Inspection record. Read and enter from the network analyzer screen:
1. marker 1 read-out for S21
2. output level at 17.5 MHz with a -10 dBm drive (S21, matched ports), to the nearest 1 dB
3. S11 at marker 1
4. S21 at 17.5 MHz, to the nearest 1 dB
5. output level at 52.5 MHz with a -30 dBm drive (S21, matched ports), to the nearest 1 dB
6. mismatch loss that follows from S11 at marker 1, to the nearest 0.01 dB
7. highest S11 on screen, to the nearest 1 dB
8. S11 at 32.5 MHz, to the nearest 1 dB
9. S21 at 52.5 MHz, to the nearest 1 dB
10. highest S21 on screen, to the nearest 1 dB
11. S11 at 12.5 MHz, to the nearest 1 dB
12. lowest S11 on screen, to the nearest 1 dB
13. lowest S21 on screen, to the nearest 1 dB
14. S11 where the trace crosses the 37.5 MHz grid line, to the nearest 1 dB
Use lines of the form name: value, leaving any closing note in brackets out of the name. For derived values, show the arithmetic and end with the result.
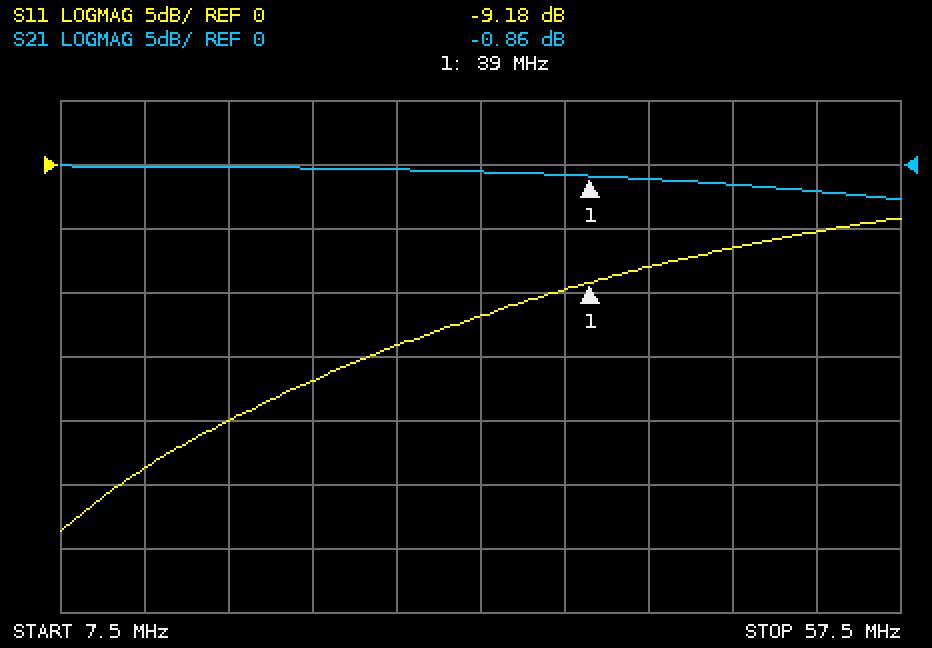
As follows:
marker 1 read-out for S21: -0.86 dB
output level at 17.5 MHz with a -10 dBm drive (S21, matched ports), to the nearest 1 dB: -10 dBm + (0 dB) = -10 dBm
S11 at marker 1: -9.18 dB
S21 at 17.5 MHz, to the nearest 1 dB: 0 dB
output level at 52.5 MHz with a -30 dBm drive (S21, matched ports), to the nearest 1 dB: -30 dBm + (-2 dB) = -32 dBm
mismatch loss that follows from S11 at marker 1, to the nearest 0.01 dB: −10 log10(1 − 10^(-9.18/10)) ≈ 0.56 dB
highest S11 on screen, to the nearest 1 dB: -4 dB
S11 at 32.5 MHz, to the nearest 1 dB: -12 dB
S21 at 52.5 MHz, to the nearest 1 dB: -2 dB
highest S21 on screen, to the nearest 1 dB: 0 dB
S11 at 12.5 MHz, to the nearest 1 dB: -24 dB
lowest S11 on screen, to the nearest 1 dB: -29 dB
lowest S21 on screen, to the nearest 1 dB: -3 dB
S11 where the trace crosses the 37.5 MHz grid line, to the nearest 1 dB: -10 dB
